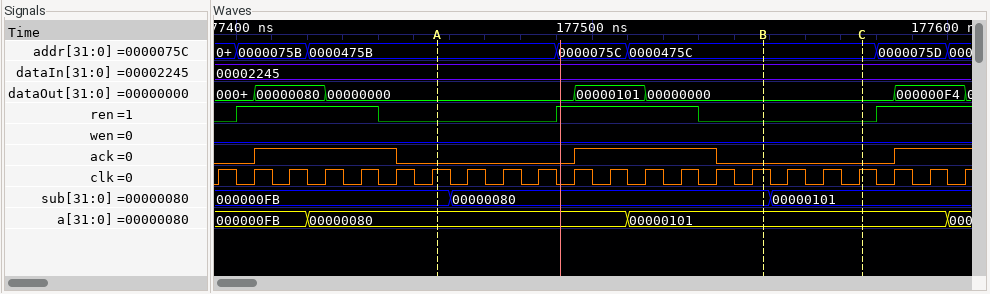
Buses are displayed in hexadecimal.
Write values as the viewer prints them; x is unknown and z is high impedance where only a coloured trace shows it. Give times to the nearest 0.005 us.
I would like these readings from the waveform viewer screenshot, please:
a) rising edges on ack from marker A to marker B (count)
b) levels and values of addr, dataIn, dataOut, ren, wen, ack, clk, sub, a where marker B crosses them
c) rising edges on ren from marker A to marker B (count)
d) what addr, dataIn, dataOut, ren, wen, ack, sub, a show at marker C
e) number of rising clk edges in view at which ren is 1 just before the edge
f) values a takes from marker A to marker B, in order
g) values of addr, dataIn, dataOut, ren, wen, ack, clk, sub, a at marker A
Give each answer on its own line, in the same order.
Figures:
1
addr=0000475C, dataIn=00002245, dataOut=00000000, ren=0, wen=0, ack=0, clk=1, sub=00000080, a=00000101
1
addr=0000475C, dataIn=00002245, dataOut=00000000, ren=0, wen=0, ack=0, sub=00000101, a=00000101
11
00000080, 00000101
addr=0000475B, dataIn=00002245, dataOut=00000000, ren=0, wen=0, ack=0, clk=1, sub=000000FB, a=00000080
